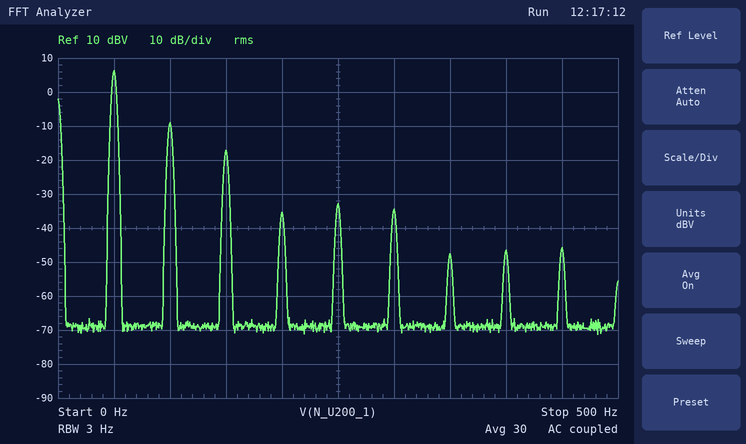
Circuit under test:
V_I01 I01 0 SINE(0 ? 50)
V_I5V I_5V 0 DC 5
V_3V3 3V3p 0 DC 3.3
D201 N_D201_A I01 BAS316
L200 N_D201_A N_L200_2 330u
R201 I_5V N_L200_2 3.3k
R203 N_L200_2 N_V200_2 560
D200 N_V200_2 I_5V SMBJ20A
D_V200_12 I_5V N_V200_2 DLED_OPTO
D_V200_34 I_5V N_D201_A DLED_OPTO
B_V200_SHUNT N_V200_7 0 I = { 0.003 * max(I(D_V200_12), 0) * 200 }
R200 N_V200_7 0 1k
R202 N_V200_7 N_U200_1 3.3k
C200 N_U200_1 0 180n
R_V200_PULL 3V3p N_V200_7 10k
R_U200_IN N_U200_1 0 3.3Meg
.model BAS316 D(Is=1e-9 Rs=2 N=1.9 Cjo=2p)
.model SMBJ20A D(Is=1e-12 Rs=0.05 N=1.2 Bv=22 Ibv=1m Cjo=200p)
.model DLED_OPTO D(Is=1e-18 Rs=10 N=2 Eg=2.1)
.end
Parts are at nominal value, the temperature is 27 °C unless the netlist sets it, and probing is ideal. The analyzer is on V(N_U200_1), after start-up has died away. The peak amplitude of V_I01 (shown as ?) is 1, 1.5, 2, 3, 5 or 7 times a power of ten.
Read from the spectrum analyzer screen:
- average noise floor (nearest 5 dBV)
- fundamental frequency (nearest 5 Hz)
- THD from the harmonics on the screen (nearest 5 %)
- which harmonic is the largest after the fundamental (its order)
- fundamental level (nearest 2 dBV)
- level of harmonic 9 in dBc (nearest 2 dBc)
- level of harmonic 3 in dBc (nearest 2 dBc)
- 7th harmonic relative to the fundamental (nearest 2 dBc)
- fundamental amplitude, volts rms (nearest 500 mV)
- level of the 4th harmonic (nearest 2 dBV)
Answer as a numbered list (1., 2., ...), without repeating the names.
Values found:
1. -70 dBV
2. 50 Hz
3. 20 %
4. 2
5. 6 dBV
6. -52 dBc
7. -24 dBc
8. -54 dBc
9. 2.0 V
10. -36 dBV
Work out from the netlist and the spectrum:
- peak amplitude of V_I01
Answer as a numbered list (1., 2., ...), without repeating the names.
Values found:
1. 5 V
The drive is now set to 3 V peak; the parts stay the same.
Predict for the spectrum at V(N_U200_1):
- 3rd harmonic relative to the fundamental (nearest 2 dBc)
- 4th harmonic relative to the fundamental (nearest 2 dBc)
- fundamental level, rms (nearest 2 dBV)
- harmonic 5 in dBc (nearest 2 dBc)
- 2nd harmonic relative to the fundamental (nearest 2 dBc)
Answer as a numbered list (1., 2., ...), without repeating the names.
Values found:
1. -32 dBc
2. -38 dBc
3. 4 dBV
4. -46 dBc
5. -26 dBc
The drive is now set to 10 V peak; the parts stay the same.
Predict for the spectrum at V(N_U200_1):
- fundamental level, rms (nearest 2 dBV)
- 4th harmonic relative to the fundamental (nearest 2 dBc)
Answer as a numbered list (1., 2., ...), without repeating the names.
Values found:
1. 10 dBV
2. -30 dBc
